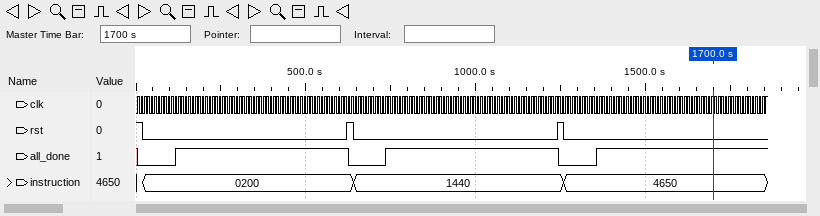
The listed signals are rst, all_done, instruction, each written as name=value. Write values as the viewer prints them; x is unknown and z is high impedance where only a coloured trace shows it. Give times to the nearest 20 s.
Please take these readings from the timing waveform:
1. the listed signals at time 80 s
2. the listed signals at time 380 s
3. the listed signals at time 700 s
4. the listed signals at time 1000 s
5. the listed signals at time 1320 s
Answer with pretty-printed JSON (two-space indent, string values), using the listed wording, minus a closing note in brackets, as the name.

{
  "the listed signals at time 80 s": "rst=0, all_done=0, instruction=0200",
  "the listed signals at time 380 s": "rst=0, all_done=1, instruction=0200",
  "the listed signals at time 700 s": "rst=0, all_done=0, instruction=1440",
  "the listed signals at time 1000 s": "rst=0, all_done=1, instruction=1440",
  "the listed signals at time 1320 s": "rst=0, all_done=0, instruction=4650"
}
